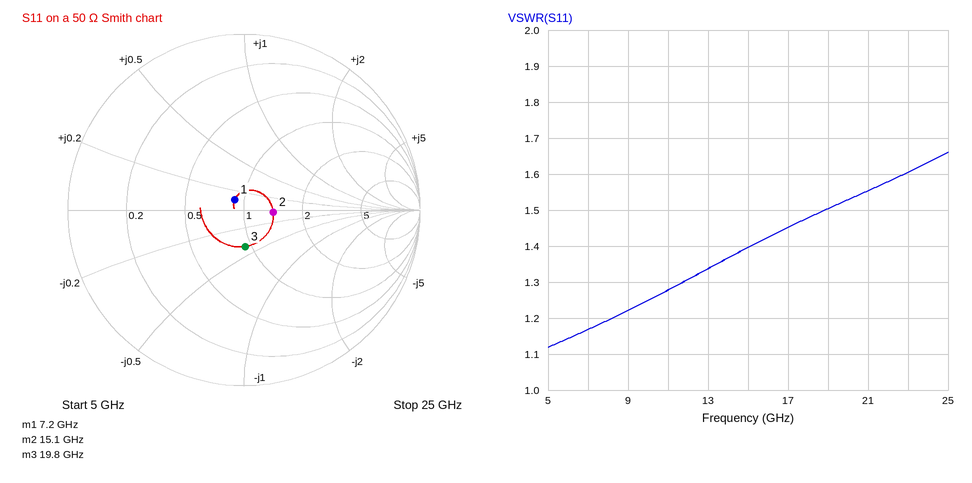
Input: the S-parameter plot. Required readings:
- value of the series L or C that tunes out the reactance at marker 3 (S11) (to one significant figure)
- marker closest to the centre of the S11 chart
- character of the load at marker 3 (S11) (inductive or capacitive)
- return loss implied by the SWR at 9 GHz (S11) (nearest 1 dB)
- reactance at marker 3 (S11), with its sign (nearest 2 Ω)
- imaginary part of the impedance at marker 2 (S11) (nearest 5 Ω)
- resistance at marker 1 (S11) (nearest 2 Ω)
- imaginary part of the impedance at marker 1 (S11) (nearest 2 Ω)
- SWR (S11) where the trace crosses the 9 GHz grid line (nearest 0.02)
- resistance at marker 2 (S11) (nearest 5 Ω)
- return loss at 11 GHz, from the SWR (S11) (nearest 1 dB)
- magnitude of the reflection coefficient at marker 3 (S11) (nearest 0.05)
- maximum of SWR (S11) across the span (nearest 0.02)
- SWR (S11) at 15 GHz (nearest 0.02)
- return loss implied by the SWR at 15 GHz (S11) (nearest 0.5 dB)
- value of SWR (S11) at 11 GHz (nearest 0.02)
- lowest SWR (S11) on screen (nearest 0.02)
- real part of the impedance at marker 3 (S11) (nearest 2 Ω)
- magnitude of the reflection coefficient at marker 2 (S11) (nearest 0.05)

200 pH
marker 1
capacitive
20 dB
-20 Ω
0 Ω
44 Ω
+6 Ω
1.22
70 Ω
18 dB
0.20
1.66
1.40
15.5 dB
1.28
1.12
46 Ω
0.15
